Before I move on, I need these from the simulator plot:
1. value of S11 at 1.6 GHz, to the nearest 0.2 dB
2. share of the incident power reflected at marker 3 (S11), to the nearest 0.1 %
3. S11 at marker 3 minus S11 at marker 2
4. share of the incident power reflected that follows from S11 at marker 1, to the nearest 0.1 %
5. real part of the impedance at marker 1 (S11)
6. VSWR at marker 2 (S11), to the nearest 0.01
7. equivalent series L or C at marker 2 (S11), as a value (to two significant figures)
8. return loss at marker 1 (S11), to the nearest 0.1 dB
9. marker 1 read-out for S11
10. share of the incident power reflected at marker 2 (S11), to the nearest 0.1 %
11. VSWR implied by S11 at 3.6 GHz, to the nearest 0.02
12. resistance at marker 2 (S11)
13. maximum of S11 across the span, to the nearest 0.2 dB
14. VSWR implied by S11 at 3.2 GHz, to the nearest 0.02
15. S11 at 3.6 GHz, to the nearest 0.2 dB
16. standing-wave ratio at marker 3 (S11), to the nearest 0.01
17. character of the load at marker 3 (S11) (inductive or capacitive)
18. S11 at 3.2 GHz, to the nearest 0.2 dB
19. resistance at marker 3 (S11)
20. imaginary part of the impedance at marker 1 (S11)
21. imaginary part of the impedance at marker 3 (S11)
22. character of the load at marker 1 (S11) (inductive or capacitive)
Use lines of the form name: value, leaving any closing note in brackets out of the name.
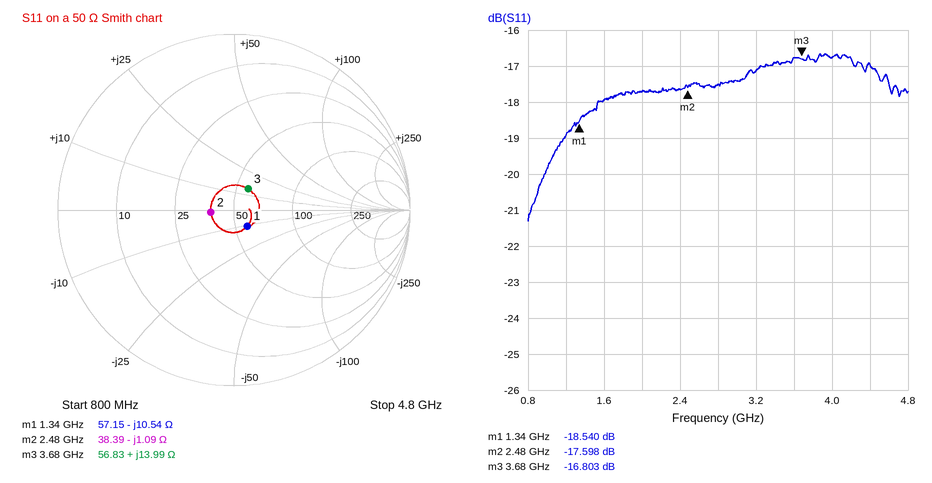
value of S11 at 1.6 GHz, to the nearest 0.2 dB: -18.0 dB
share of the incident power reflected at marker 3 (S11), to the nearest 0.1 %: 2.1 %
S11 at marker 3 minus S11 at marker 2: 0.795 dB
share of the incident power reflected that follows from S11 at marker 1, to the nearest 0.1 %: 1.4 %
real part of the impedance at marker 1: 57.15 Ω
VSWR at marker 2 (S11), to the nearest 0.01: 1.30
equivalent series L or C at marker 2 (S11), as a value: 59 pF
return loss at marker 1 (S11), to the nearest 0.1 dB: 18.5 dB
marker 1 read-out for S11: -18.540 dB
share of the incident power reflected at marker 2 (S11), to the nearest 0.1 %: 1.7 %
VSWR implied by S11 at 3.6 GHz, to the nearest 0.02: 1.34
resistance at marker 2: 38.39 Ω
maximum of S11 across the span, to the nearest 0.2 dB: -16.6 dB
VSWR implied by S11 at 3.2 GHz, to the nearest 0.02: 1.32
S11 at 3.6 GHz, to the nearest 0.2 dB: -16.8 dB
standing-wave ratio at marker 3 (S11), to the nearest 0.01: 1.34
character of the load at marker 3 (S11): inductive
S11 at 3.2 GHz, to the nearest 0.2 dB: -17.2 dB
resistance at marker 3: 56.83 Ω
imaginary part of the impedance at marker 1: -10.54 Ω
imaginary part of the impedance at marker 3: +13.99 Ω
character of the load at marker 1 (S11): capacitive
